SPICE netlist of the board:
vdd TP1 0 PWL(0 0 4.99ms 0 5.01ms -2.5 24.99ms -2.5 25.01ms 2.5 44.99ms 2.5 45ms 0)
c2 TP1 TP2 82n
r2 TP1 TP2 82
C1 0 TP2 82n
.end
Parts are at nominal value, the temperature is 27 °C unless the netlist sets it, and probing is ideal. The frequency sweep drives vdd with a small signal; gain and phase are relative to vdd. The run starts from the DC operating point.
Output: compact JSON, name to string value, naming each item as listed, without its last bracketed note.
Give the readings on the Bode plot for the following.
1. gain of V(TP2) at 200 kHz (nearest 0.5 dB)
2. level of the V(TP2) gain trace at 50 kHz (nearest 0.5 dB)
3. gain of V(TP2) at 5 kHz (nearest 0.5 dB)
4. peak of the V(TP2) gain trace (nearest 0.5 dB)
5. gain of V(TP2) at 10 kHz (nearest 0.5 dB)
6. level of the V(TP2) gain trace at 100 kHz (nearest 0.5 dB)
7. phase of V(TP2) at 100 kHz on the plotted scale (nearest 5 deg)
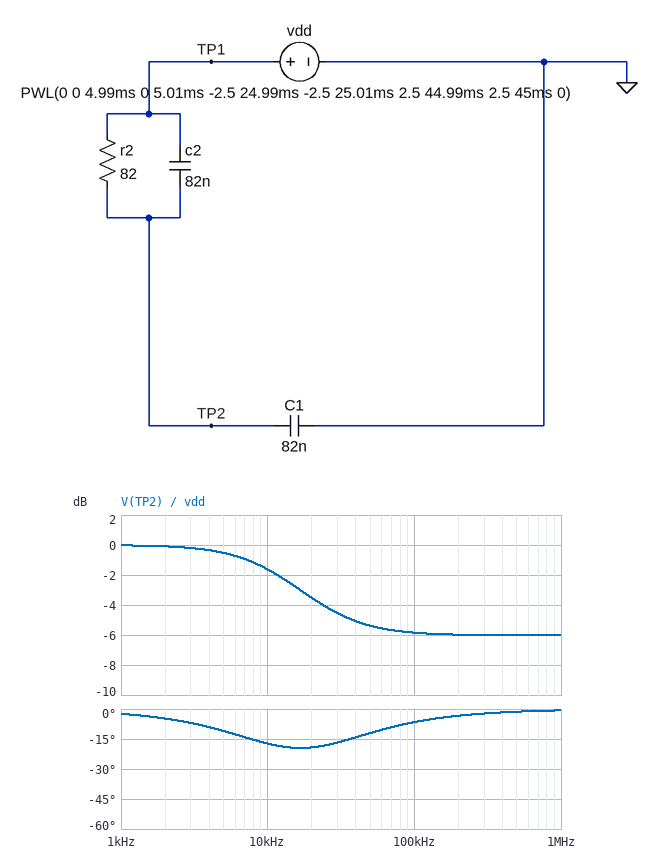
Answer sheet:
{"gain of V(TP2) at 200 kHz": "-6.0 dB", "level of the V(TP2) gain trace at 50 kHz": "-5.5 dB", "gain of V(TP2) at 5 kHz": "-0.5 dB", "peak of the V(TP2) gain trace": "0 dB", "gain of V(TP2) at 10 kHz": "-1.5 dB", "level of the V(TP2) gain trace at 100 kHz": "-6.0 dB", "phase of V(TP2) at 100 kHz on the plotted scale": "-5 deg"}
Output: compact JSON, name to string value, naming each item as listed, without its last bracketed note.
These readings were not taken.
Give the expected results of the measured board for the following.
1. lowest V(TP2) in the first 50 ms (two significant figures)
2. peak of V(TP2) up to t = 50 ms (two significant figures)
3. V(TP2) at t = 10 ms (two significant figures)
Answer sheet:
{"lowest V(TP2) in the first 50 ms": "-2.5 V", "peak of V(TP2) up to t = 50 ms": "2.5 V", "V(TP2) at t = 10 ms": "-2.5 V"}
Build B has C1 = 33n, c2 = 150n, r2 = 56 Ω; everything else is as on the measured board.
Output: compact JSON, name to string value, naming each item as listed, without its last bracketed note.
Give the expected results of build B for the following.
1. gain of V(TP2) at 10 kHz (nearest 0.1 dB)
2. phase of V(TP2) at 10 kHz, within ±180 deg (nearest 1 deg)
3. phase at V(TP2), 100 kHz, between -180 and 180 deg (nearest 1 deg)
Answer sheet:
{"gain of V(TP2) at 10 kHz": "-0.4 dB", "phase of V(TP2) at 10 kHz, within ±180 deg": "-5 deg", "phase at V(TP2), 100 kHz, between -180 and 180 deg": "-2 deg"}
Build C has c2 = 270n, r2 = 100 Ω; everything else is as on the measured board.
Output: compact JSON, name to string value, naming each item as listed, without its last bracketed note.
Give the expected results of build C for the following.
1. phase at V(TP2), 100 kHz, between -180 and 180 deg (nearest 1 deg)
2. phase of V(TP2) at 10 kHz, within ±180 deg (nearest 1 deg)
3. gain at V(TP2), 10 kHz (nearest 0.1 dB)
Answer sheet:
{"phase at V(TP2), 100 kHz, between -180 and 180 deg": "-1 deg", "phase of V(TP2) at 10 kHz, within ±180 deg": "-6 deg", "gain at V(TP2), 10 kHz": "-1.8 dB"}
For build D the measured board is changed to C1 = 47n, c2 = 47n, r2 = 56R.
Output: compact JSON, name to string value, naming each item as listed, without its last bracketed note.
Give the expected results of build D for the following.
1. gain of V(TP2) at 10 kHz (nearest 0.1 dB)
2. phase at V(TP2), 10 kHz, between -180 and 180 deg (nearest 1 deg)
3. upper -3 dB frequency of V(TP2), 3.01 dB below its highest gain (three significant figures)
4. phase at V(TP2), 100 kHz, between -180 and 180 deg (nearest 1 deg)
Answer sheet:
{"gain of V(TP2) at 10 kHz": "-0.3 dB", "phase at V(TP2), 10 kHz, between -180 and 180 deg": "-9 deg", "upper -3 dB frequency of V(TP2), 3.01 dB below its highest gain": "42.8 kHz", "phase at V(TP2), 100 kHz, between -180 and 180 deg": "-14 deg"}
